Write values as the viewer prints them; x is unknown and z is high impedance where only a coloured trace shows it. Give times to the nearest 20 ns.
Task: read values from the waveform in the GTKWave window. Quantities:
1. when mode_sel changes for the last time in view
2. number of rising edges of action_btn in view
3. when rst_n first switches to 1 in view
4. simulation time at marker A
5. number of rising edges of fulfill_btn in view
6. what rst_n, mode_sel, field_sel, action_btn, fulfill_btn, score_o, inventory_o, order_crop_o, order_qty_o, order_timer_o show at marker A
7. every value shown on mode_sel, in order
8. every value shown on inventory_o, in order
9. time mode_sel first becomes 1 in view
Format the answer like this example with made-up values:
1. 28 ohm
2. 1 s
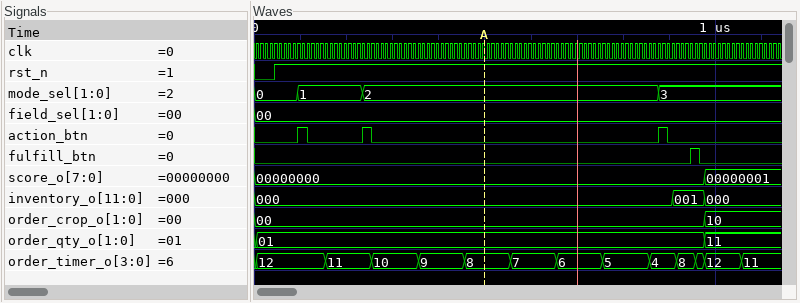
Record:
1. 880 ns
2. 3
3. 40 ns
4. 500 ns
5. 1
6. rst_n=1, mode_sel=2, field_sel=00, action_btn=0, fulfill_btn=0, score_o=00000000, inventory_o=000, order_crop_o=00, order_qty_o=01, order_timer_o=8
7. 0, 1, 2, 3
8. 000, 001, 000
9. 100 ns
